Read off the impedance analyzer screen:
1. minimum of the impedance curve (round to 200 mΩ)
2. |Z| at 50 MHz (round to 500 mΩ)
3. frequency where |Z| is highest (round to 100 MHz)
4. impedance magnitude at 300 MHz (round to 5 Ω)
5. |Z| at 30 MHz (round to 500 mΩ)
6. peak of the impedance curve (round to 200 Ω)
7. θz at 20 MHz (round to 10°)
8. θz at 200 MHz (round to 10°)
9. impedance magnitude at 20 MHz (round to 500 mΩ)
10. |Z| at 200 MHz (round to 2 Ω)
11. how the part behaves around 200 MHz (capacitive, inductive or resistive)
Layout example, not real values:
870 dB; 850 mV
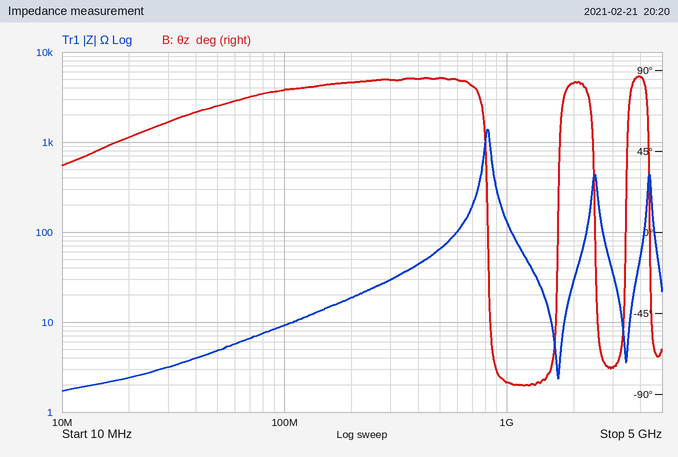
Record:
1.8 Ω; 5.0 Ω; 800 MHz; 30 Ω; 3.0 Ω; 1.4 kΩ; 50°; 80°; 2.5 Ω; 18 Ω; inductive
